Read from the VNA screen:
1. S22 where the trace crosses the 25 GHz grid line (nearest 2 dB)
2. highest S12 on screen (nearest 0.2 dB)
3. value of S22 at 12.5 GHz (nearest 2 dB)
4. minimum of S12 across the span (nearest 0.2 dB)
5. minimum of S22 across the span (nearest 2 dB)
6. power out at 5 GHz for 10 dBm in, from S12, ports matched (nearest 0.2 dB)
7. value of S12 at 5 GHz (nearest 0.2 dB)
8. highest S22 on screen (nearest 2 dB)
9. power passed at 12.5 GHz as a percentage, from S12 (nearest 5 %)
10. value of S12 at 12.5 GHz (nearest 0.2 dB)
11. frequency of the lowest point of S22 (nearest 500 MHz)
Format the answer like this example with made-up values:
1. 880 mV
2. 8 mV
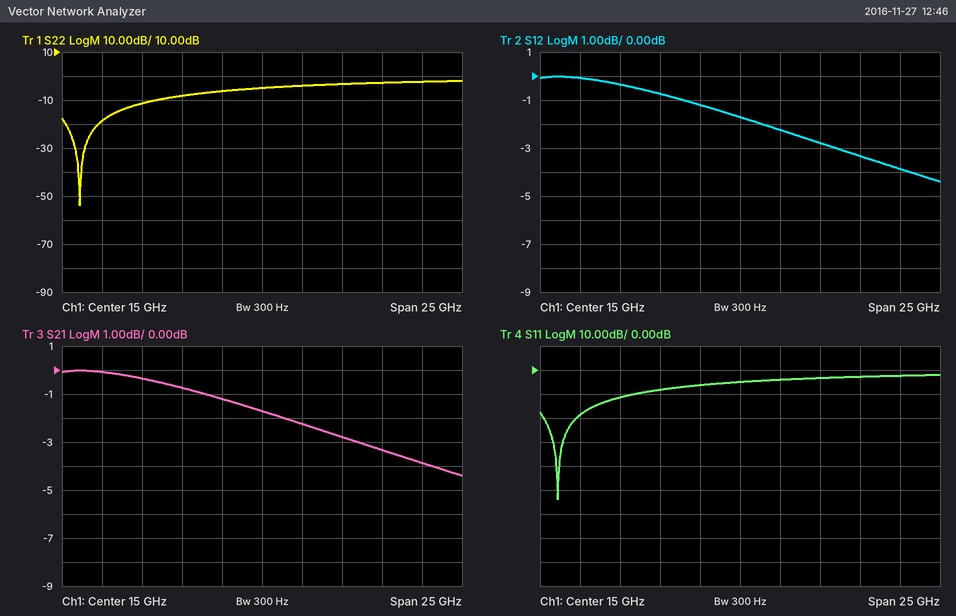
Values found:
1. -2 dB
2. 0.0 dB
3. -6 dB
4. -4.4 dB
5. -54 dB
6. 10.0 dBm
7. 0.0 dB
8. -2 dB
9. 75 %
10. -1.2 dB
11. 3.5 GHz
